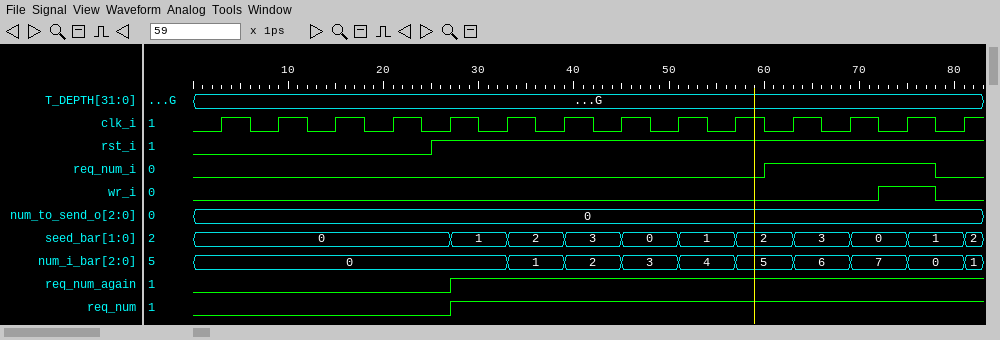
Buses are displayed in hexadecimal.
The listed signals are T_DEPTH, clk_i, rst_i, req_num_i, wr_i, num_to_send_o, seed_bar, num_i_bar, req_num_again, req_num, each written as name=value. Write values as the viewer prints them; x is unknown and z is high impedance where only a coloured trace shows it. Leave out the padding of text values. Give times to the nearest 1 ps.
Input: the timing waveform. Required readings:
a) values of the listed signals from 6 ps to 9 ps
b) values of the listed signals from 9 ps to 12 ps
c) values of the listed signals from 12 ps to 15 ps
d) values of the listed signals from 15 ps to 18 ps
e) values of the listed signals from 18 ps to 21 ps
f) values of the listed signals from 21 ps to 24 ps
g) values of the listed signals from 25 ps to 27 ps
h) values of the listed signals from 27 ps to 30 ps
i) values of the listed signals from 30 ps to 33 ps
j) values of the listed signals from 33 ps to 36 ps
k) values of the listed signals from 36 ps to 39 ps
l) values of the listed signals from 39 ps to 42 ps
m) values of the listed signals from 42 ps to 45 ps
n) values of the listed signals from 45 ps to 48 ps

T_DEPTH=G, clk_i=0, rst_i=0, req_num_i=0, wr_i=0, num_to_send_o=0, seed_bar=0, num_i_bar=0, req_num_again=0, req_num=0
T_DEPTH=G, clk_i=1, rst_i=0, req_num_i=0, wr_i=0, num_to_send_o=0, seed_bar=0, num_i_bar=0, req_num_again=0, req_num=0
T_DEPTH=G, clk_i=0, rst_i=0, req_num_i=0, wr_i=0, num_to_send_o=0, seed_bar=0, num_i_bar=0, req_num_again=0, req_num=0
T_DEPTH=G, clk_i=1, rst_i=0, req_num_i=0, wr_i=0, num_to_send_o=0, seed_bar=0, num_i_bar=0, req_num_again=0, req_num=0
T_DEPTH=G, clk_i=0, rst_i=0, req_num_i=0, wr_i=0, num_to_send_o=0, seed_bar=0, num_i_bar=0, req_num_again=0, req_num=0
T_DEPTH=G, clk_i=1, rst_i=0, req_num_i=0, wr_i=0, num_to_send_o=0, seed_bar=0, num_i_bar=0, req_num_again=0, req_num=0
T_DEPTH=G, clk_i=0, rst_i=1, req_num_i=0, wr_i=0, num_to_send_o=0, seed_bar=0, num_i_bar=0, req_num_again=0, req_num=0
T_DEPTH=G, clk_i=1, rst_i=1, req_num_i=0, wr_i=0, num_to_send_o=0, seed_bar=1, num_i_bar=0, req_num_again=1, req_num=1
T_DEPTH=G, clk_i=0, rst_i=1, req_num_i=0, wr_i=0, num_to_send_o=0, seed_bar=1, num_i_bar=0, req_num_again=1, req_num=1
T_DEPTH=G, clk_i=1, rst_i=1, req_num_i=0, wr_i=0, num_to_send_o=0, seed_bar=2, num_i_bar=1, req_num_again=1, req_num=1
T_DEPTH=G, clk_i=0, rst_i=1, req_num_i=0, wr_i=0, num_to_send_o=0, seed_bar=2, num_i_bar=1, req_num_again=1, req_num=1
T_DEPTH=G, clk_i=1, rst_i=1, req_num_i=0, wr_i=0, num_to_send_o=0, seed_bar=3, num_i_bar=2, req_num_again=1, req_num=1
T_DEPTH=G, clk_i=0, rst_i=1, req_num_i=0, wr_i=0, num_to_send_o=0, seed_bar=3, num_i_bar=2, req_num_again=1, req_num=1
T_DEPTH=G, clk_i=1, rst_i=1, req_num_i=0, wr_i=0, num_to_send_o=0, seed_bar=0, num_i_bar=3, req_num_again=1, req_num=1
